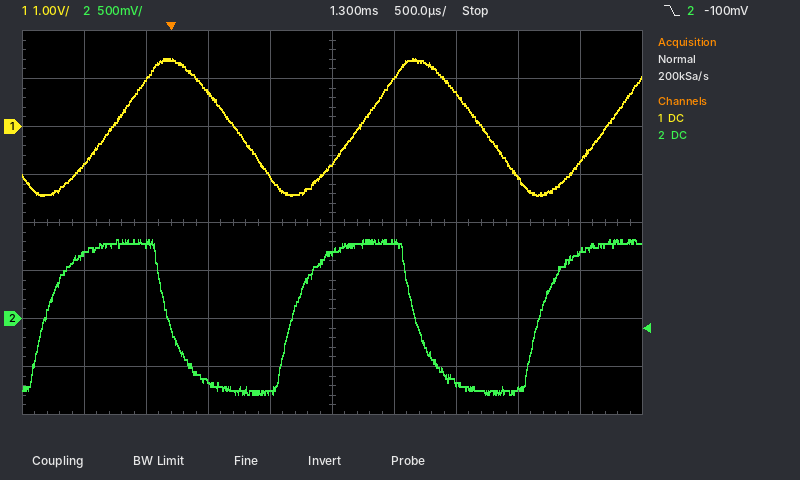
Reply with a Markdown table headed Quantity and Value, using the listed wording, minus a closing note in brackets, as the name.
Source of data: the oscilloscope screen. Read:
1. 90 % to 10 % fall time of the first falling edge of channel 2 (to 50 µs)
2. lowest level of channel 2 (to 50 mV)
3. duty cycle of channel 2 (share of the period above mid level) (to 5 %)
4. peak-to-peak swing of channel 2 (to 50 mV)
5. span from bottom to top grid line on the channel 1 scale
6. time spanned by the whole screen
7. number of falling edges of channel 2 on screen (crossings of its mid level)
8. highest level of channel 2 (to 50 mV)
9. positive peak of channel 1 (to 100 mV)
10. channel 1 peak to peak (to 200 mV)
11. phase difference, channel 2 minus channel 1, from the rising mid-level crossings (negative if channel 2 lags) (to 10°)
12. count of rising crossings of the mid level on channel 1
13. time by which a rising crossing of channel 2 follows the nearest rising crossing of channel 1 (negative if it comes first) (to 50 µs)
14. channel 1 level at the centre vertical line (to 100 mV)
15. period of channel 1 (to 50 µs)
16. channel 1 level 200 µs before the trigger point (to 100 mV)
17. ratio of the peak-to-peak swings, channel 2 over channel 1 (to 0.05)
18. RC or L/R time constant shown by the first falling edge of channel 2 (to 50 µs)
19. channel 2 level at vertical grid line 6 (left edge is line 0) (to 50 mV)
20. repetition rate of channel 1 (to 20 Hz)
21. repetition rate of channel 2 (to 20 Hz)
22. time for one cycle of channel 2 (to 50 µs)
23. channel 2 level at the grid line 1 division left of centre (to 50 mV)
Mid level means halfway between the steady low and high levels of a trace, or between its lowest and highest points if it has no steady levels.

| Quantity | Value |
|---|---|
| 90 % to 10 % fall time of the first falling edge of channel 2 | 350 µs |
| lowest level of channel 2 | -800 mV |
| duty cycle of channel 2 (share of the period above mid level) | 50 % |
| peak-to-peak swing of channel 2 | 1.60 V |
| span from bottom to top grid line on the channel 1 scale | 8 V |
| time spanned by the whole screen | 5 ms |
| number of falling edges of channel 2 on screen | 2 |
| highest level of channel 2 | 800 mV |
| positive peak of channel 1 | 1.4 V |
| channel 1 peak to peak | 2.8 V |
| phase difference, channel 2 minus channel 1, from the rising mid-level crossings (negative if channel 2 lags) | +100° |
| count of rising crossings of the mid level on channel 1 | 3 |
| time by which a rising crossing of channel 2 follows the nearest rising crossing of channel 1 (negative if it comes first) | -550 µs |
| channel 1 level at the centre vertical line | -800 mV |
| period of channel 1 | 2.00 ms |
| channel 1 level 200 µs before the trigger point | 1.0 V |
| ratio of the peak-to-peak swings, channel 2 over channel 1 | 0.55 |
| RC or L/R time constant shown by the first falling edge of channel 2 | 150 µs |
| channel 2 level at vertical grid line 6 (left edge is line 0) | 800 mV |
| repetition rate of channel 1 | 500 Hz |
| repetition rate of channel 2 | 500 Hz |
| time for one cycle of channel 2 | 2.00 ms |
| channel 2 level at the grid line 1 division left of centre | -750 mV |
